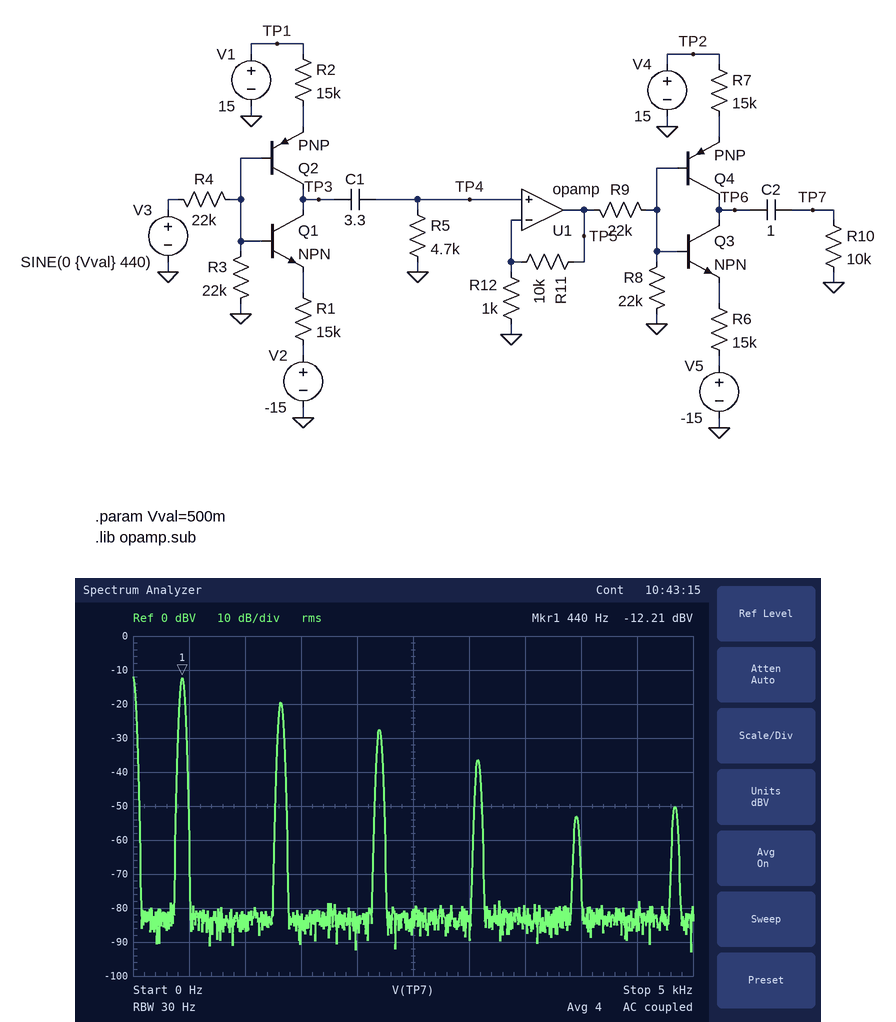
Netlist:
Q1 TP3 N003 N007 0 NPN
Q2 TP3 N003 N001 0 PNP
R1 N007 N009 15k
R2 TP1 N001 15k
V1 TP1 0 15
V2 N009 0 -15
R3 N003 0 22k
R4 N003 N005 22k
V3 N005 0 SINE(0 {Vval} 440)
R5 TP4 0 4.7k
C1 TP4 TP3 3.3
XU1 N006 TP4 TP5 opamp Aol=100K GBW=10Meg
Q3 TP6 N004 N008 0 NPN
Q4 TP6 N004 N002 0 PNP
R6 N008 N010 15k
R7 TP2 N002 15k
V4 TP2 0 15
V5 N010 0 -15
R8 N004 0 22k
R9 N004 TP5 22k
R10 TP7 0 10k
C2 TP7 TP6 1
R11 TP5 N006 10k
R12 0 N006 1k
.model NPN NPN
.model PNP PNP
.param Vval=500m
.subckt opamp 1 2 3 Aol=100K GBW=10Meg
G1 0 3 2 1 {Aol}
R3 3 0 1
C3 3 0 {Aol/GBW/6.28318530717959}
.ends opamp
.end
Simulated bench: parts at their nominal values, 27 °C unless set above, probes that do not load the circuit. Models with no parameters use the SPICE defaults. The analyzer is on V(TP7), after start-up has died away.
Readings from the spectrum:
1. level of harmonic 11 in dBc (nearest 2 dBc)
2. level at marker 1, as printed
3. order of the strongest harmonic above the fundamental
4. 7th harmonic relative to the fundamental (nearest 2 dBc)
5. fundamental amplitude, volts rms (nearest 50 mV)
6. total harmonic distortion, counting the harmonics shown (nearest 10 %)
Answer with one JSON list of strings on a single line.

["-38 dBc", "-12.21 dBV", "3", "-24 dBc", "250 mV", "50 %"]
